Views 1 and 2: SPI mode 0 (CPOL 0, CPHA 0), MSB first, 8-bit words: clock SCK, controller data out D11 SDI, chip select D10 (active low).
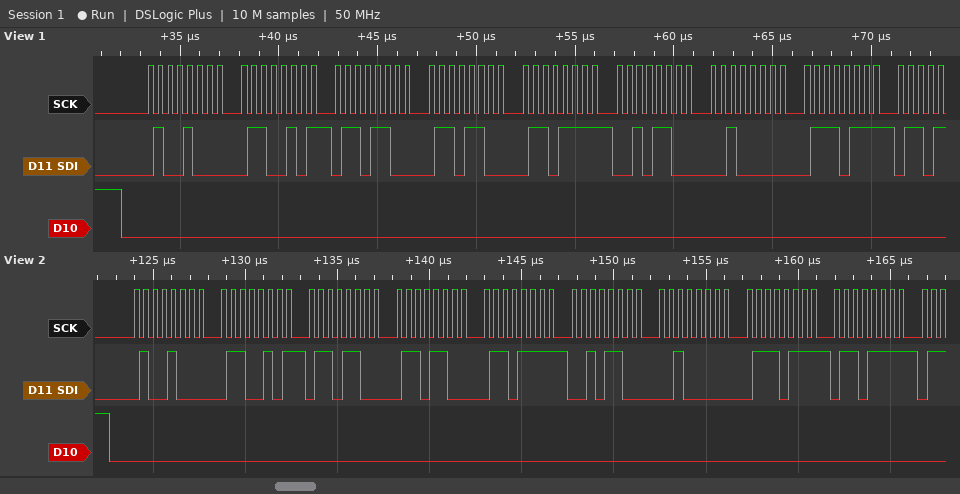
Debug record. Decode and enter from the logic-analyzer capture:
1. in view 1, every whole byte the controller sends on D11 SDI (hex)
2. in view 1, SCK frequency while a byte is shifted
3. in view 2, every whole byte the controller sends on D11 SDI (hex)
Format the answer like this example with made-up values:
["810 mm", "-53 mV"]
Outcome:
["0x48 0x65 0x6C 0x6C 0x6F 0x2C 0x20 0x77", "2 MHz", "0x48 0x65 0x6C 0x6C 0x6F 0x2C 0x20 0x77 0x6F"]
